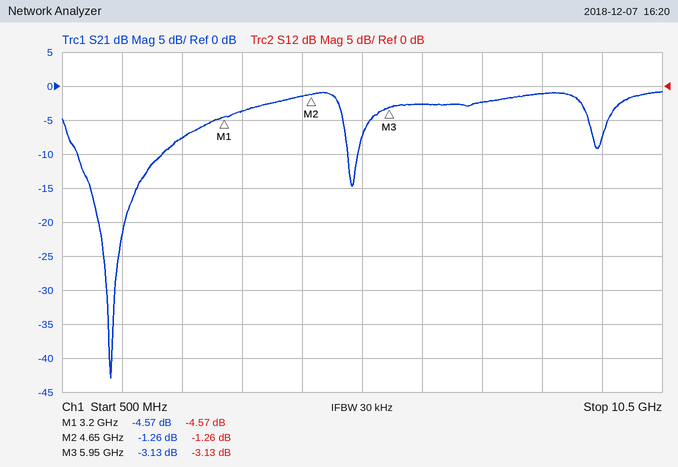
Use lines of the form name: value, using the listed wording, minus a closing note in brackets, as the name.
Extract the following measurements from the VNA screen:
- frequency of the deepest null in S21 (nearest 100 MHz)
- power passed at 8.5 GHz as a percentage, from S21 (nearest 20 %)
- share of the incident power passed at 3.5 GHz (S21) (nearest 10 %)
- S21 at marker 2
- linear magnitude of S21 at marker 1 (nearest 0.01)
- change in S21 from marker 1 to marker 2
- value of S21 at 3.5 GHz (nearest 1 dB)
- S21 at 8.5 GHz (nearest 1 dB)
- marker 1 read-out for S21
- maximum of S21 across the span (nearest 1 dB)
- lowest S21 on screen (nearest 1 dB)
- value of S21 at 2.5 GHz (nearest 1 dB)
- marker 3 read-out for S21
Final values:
frequency of the deepest null in S21: 1.3 GHz
power passed at 8.5 GHz as a percentage, from S21: 80 %
share of the incident power passed at 3.5 GHz (S21): 40 %
S21 at marker 2: -1.26 dB
linear magnitude of S21 at marker 1: 0.59
change in S21 from marker 1 to marker 2: 3.31 dB
value of S21 at 3.5 GHz: -4 dB
S21 at 8.5 GHz: -1 dB
marker 1 read-out for S21: -4.57 dB
maximum of S21 across the span: -1 dB
lowest S21 on screen: -43 dB
value of S21 at 2.5 GHz: -8 dB
marker 3 read-out for S21: -3.13 dB
